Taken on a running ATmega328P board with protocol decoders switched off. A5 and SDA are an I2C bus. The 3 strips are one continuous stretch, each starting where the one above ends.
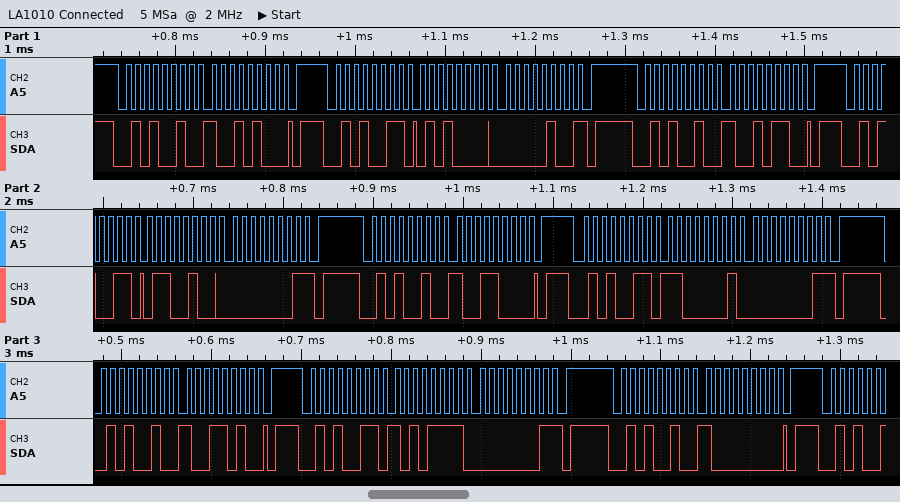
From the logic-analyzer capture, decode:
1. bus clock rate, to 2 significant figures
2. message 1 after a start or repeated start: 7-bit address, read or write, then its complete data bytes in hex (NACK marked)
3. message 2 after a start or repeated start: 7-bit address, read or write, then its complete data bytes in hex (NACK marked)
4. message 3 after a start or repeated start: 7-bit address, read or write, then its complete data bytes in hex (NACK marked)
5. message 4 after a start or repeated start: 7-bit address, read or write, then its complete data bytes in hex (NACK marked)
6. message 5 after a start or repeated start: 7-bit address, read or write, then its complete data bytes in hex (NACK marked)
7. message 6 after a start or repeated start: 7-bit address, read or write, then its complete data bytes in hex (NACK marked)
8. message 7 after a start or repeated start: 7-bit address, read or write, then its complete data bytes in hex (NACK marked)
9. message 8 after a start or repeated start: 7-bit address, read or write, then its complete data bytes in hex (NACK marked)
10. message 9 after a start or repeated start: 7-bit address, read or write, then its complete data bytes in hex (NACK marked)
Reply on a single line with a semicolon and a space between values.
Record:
100 kHz; 0x29 write: 94; 0x29 read: 50 04 NACK; 0x29 write: 96; 0x29 read: 64 01 NACK; 0x29 write: 98; 0x29 read: C1 01 NACK; 0x29 write: 9A; 0x29 read: AF 01 NACK; 0x29 write: 80
